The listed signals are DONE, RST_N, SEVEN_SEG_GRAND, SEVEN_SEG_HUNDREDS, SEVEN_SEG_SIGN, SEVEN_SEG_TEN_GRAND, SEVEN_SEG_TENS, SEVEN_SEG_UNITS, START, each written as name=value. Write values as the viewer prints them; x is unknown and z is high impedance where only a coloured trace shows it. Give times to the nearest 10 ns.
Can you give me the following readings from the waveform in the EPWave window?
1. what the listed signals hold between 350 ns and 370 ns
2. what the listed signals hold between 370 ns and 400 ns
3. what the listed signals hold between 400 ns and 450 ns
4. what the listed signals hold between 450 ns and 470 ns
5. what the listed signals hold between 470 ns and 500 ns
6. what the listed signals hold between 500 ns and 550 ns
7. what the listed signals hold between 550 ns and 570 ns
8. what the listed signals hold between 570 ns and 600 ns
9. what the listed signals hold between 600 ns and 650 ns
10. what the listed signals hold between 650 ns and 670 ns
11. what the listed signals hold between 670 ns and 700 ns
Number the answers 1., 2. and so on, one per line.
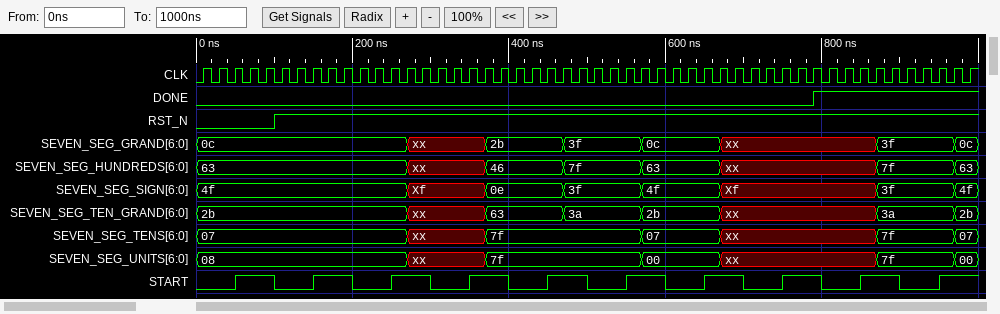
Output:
1. DONE=0, RST_N=1, SEVEN_SEG_GRAND=xx, SEVEN_SEG_HUNDREDS=xx, SEVEN_SEG_SIGN=Xf, SEVEN_SEG_TEN_GRAND=xx, SEVEN_SEG_TENS=xx, SEVEN_SEG_UNITS=xx, START=1
2. DONE=0, RST_N=1, SEVEN_SEG_GRAND=2b, SEVEN_SEG_HUNDREDS=46, SEVEN_SEG_SIGN=0e, SEVEN_SEG_TEN_GRAND=63, SEVEN_SEG_TENS=7f, SEVEN_SEG_UNITS=7f, START=1
3. DONE=0, RST_N=1, SEVEN_SEG_GRAND=2b, SEVEN_SEG_HUNDREDS=46, SEVEN_SEG_SIGN=0e, SEVEN_SEG_TEN_GRAND=63, SEVEN_SEG_TENS=7f, SEVEN_SEG_UNITS=7f, START=0
4. DONE=0, RST_N=1, SEVEN_SEG_GRAND=2b, SEVEN_SEG_HUNDREDS=46, SEVEN_SEG_SIGN=0e, SEVEN_SEG_TEN_GRAND=63, SEVEN_SEG_TENS=7f, SEVEN_SEG_UNITS=7f, START=1
5. DONE=0, RST_N=1, SEVEN_SEG_GRAND=3f, SEVEN_SEG_HUNDREDS=7f, SEVEN_SEG_SIGN=3f, SEVEN_SEG_TEN_GRAND=3a, SEVEN_SEG_TENS=7f, SEVEN_SEG_UNITS=7f, START=1
6. DONE=0, RST_N=1, SEVEN_SEG_GRAND=3f, SEVEN_SEG_HUNDREDS=7f, SEVEN_SEG_SIGN=3f, SEVEN_SEG_TEN_GRAND=3a, SEVEN_SEG_TENS=7f, SEVEN_SEG_UNITS=7f, START=0
7. DONE=0, RST_N=1, SEVEN_SEG_GRAND=3f, SEVEN_SEG_HUNDREDS=7f, SEVEN_SEG_SIGN=3f, SEVEN_SEG_TEN_GRAND=3a, SEVEN_SEG_TENS=7f, SEVEN_SEG_UNITS=7f, START=1
8. DONE=0, RST_N=1, SEVEN_SEG_GRAND=0c, SEVEN_SEG_HUNDREDS=63, SEVEN_SEG_SIGN=4f, SEVEN_SEG_TEN_GRAND=2b, SEVEN_SEG_TENS=07, SEVEN_SEG_UNITS=00, START=1
9. DONE=0, RST_N=1, SEVEN_SEG_GRAND=0c, SEVEN_SEG_HUNDREDS=63, SEVEN_SEG_SIGN=4f, SEVEN_SEG_TEN_GRAND=2b, SEVEN_SEG_TENS=07, SEVEN_SEG_UNITS=00, START=0
10. DONE=0, RST_N=1, SEVEN_SEG_GRAND=0c, SEVEN_SEG_HUNDREDS=63, SEVEN_SEG_SIGN=4f, SEVEN_SEG_TEN_GRAND=2b, SEVEN_SEG_TENS=07, SEVEN_SEG_UNITS=00, START=1
11. DONE=0, RST_N=1, SEVEN_SEG_GRAND=xx, SEVEN_SEG_HUNDREDS=xx, SEVEN_SEG_SIGN=Xf, SEVEN_SEG_TEN_GRAND=xx, SEVEN_SEG_TENS=xx, SEVEN_SEG_UNITS=xx, START=1
